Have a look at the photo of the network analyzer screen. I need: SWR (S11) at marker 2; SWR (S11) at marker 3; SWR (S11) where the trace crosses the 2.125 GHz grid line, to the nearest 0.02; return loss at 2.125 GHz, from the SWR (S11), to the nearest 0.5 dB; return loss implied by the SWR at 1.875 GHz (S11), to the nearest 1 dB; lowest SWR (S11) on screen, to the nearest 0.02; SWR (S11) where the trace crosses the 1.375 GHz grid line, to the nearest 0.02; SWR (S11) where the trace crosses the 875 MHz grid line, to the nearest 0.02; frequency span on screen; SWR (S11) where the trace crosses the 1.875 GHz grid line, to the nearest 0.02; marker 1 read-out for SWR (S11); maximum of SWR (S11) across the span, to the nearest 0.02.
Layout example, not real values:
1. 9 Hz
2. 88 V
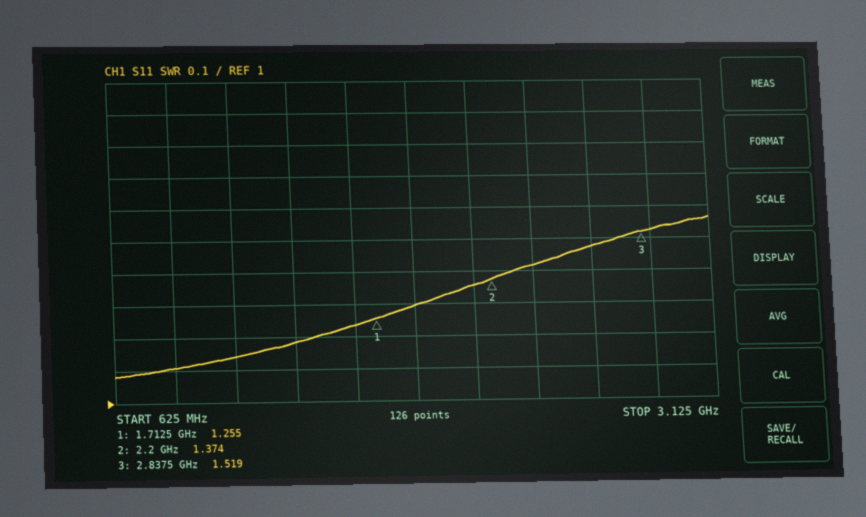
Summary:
1. 1.374
2. 1.519
3. 1.36
4. 16.5 dB
5. 18 dB
6. 1.08
7. 1.18
8. 1.10
9. 2.5 GHz
10. 1.30
11. 1.255
12. 1.56
